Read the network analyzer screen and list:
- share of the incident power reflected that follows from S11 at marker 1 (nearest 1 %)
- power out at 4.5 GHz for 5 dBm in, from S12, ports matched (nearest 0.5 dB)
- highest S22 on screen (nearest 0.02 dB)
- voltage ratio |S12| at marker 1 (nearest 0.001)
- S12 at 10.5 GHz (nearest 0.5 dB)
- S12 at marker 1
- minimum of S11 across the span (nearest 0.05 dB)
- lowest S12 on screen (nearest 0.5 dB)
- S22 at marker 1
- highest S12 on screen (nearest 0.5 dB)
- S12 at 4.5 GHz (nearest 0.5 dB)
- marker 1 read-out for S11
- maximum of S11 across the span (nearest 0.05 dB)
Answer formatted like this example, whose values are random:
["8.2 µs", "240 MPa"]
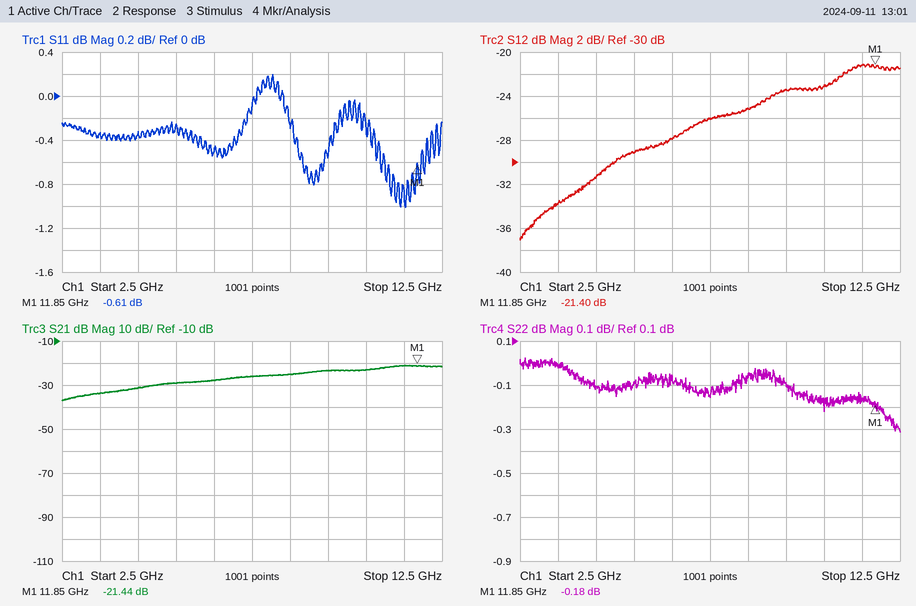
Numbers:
["87 %", "-26.5 dBm", "0.02 dB", "0.085", "-23.0 dB", "-21.40 dB", "-1.00 dB", "-37.0 dB", "-0.18 dB", "-21.0 dB", "-31.5 dB", "-0.61 dB", "0.20 dB"]
